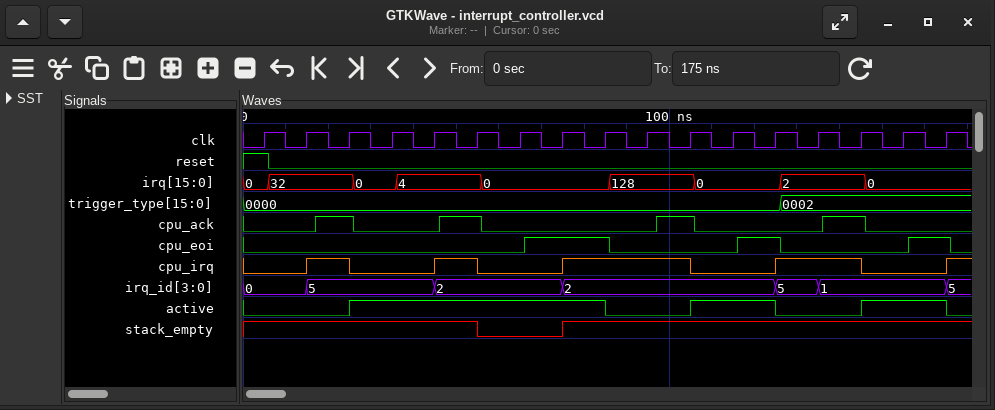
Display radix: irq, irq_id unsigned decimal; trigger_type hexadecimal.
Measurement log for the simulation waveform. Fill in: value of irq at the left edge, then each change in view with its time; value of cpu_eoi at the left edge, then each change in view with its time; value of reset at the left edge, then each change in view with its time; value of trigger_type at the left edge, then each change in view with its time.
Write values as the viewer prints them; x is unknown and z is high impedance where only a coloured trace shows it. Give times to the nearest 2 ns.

0, 32 at 6 ns, 0 at 26 ns, 4 at 36 ns, 0 at 56 ns, 128 at 86 ns, 0 at 106 ns, 2 at 126 ns, 0 at 146 ns
0, 1 at 66 ns, 0 at 86 ns, 1 at 116 ns, 0 at 126 ns, 1 at 156 ns, 0 at 166 ns
1, 0 at 6 ns
0000, 0002 at 126 ns
